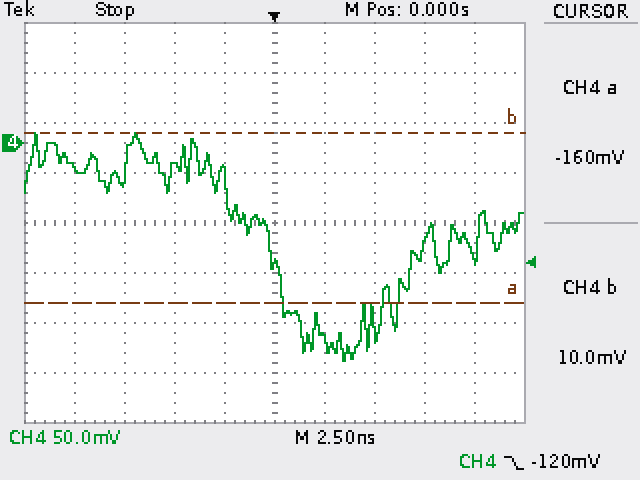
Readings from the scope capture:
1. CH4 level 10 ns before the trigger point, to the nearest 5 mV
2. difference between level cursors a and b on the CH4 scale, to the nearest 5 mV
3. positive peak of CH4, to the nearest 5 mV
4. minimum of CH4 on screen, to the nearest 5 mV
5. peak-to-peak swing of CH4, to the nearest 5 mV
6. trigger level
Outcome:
-25 mV
170 mV
10 mV
-220 mV
230 mV
-120 mV
